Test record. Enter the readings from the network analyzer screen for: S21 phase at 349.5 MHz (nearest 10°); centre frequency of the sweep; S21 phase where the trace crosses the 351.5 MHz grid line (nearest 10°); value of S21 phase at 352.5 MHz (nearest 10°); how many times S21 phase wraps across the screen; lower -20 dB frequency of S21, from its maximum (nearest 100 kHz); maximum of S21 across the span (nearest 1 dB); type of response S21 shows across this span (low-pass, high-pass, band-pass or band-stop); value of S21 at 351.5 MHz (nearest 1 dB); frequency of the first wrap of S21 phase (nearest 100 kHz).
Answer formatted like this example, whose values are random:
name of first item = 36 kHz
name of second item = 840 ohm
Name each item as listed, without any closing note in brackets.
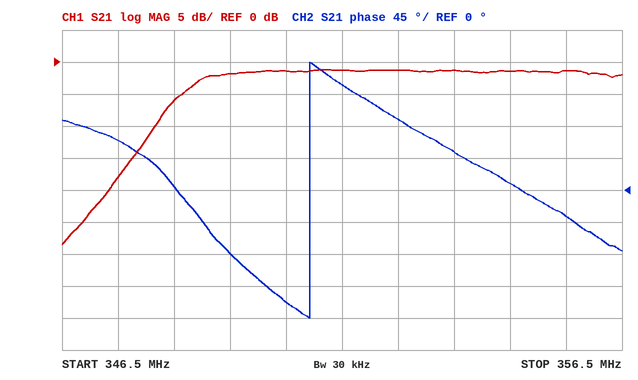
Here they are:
S21 phase at 349.5 MHz = -90°
centre frequency of the sweep = 351.5 MHz
S21 phase where the trace crosses the 351.5 MHz grid line = 150°
value of S21 phase at 352.5 MHz = 100°
how many times S21 phase wraps across the screen = 1
lower -20 dB frequency of S21, from its maximum = 347.2 MHz
maximum of S21 across the span = -1 dB
type of response S21 shows across this span = high-pass
value of S21 at 351.5 MHz = -1 dB
frequency of the first wrap of S21 phase = 350.9 MHz
